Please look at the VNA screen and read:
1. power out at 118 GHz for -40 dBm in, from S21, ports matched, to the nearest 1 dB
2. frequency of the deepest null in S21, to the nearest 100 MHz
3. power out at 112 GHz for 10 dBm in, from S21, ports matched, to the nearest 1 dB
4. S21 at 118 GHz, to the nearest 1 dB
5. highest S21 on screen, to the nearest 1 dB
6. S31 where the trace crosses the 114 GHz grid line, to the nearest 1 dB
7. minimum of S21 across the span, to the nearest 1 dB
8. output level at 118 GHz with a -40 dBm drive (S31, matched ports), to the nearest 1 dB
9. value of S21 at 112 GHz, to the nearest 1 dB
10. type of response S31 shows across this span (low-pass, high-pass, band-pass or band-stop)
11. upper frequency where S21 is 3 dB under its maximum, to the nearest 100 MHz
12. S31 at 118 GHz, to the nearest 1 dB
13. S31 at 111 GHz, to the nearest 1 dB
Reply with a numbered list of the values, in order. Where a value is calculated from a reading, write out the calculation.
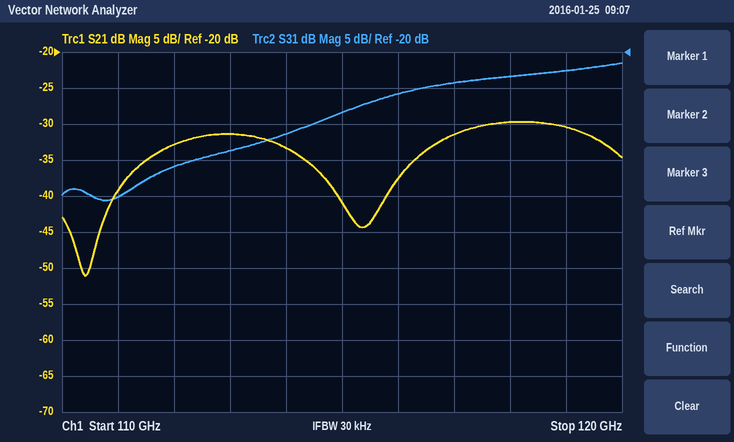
1. -40 dBm + (-30 dB) = -70 dBm
2. 110.4 GHz
3. 10 dBm + (-33 dB) = -23 dBm
4. -30 dB
5. -30 dB
6. -31 dB
7. -51 dB
8. -40 dBm + (-23 dB) = -63 dBm
9. -33 dB
10. high-pass
11. 119.7 GHz
12. -23 dB
13. -40 dB
